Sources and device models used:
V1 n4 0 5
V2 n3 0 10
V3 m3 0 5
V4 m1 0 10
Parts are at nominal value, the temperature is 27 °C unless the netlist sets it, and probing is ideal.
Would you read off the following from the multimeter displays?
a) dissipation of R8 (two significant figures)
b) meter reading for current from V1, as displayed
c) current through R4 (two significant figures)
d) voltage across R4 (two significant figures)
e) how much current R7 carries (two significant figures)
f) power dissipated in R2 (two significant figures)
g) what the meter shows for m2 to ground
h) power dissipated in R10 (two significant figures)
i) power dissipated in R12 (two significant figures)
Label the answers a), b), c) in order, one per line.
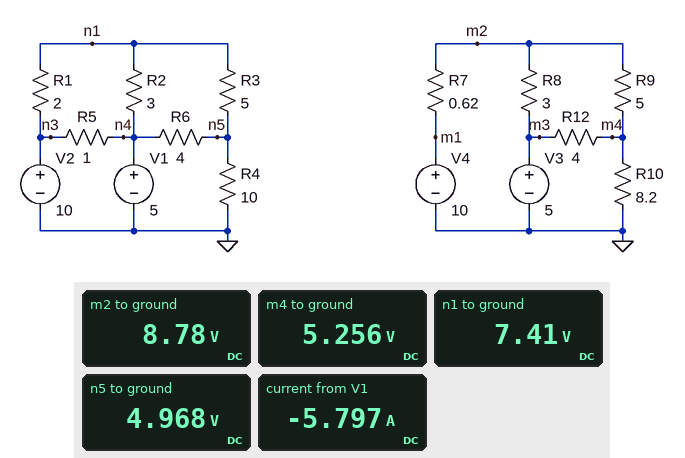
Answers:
a) 4.8 W
b) -5.797 A
c) 500 mA
d) 5.0 V
e) 2.0 A
f) 1.9 W
g) 8.78 V
h) 3.4 W
i) 16 mW
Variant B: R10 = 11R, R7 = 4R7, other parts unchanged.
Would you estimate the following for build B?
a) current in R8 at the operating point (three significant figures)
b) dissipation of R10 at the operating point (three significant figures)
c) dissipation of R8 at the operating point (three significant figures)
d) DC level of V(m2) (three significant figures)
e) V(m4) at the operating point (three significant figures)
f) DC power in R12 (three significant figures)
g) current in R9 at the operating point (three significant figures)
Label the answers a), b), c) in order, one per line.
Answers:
a) 444 mA
b) 1.97 W
c) 592 mW
d) 6.33 V
e) 4.65 V
f) 30.2 mW
g) 336 mA
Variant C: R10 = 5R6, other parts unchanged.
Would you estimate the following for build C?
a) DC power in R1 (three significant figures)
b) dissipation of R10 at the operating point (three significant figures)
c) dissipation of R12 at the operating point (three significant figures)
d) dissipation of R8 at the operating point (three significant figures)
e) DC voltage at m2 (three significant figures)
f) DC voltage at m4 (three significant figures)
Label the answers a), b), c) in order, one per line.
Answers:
a) 3.35 W
b) 4.06 W
c) 13.4 mW
d) 4.65 W
e) 8.74 V
f) 4.77 V
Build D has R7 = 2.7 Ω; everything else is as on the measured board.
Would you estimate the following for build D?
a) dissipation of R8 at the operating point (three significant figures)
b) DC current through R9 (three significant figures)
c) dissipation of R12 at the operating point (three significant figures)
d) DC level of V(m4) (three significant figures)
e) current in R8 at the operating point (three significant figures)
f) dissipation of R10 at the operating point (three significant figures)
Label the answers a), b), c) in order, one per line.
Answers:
a) 1.29 W
b) 469 mA
c) 35.9 mW
d) 4.62 V
e) 655 mA
f) 2.60 W
